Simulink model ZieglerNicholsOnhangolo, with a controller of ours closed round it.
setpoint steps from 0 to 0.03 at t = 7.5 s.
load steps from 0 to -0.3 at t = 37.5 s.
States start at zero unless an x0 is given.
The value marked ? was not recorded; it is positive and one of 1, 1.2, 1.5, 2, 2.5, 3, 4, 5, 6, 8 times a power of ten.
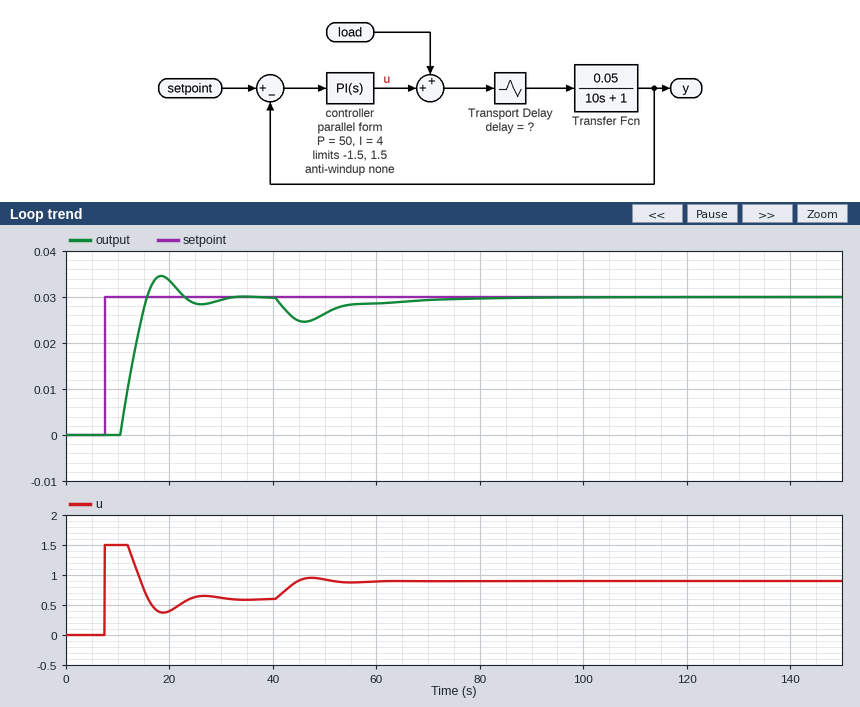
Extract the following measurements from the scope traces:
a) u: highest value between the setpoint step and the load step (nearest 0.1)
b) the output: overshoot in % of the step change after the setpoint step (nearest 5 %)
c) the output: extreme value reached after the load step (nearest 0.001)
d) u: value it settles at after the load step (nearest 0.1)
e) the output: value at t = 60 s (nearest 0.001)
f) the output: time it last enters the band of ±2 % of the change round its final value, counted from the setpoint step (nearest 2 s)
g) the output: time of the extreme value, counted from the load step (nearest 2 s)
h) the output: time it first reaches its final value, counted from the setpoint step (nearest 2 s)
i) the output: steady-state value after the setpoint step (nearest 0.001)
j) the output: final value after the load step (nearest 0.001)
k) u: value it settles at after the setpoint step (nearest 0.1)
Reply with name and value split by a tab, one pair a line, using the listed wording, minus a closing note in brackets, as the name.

u: highest value between the setpoint step and the load step	1.5
the output: overshoot in % of the step change after the setpoint step	15 %
the output: extreme value reached after the load step	0.025
u: value it settles at after the load step	0.9
the output: value at t = 60 s	0.029
the output: time it last enters the band of ±2 % of the change round its final value, counted from the setpoint step	22 s
the output: time of the extreme value, counted from the load step	8 s
the output: time it first reaches its final value, counted from the setpoint step	8 s
the output: steady-state value after the setpoint step	0.030
the output: final value after the load step	0.030
u: value it settles at after the setpoint step	0.6
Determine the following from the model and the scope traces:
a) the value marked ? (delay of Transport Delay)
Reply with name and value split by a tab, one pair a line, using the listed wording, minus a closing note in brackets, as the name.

the value marked ?	3
